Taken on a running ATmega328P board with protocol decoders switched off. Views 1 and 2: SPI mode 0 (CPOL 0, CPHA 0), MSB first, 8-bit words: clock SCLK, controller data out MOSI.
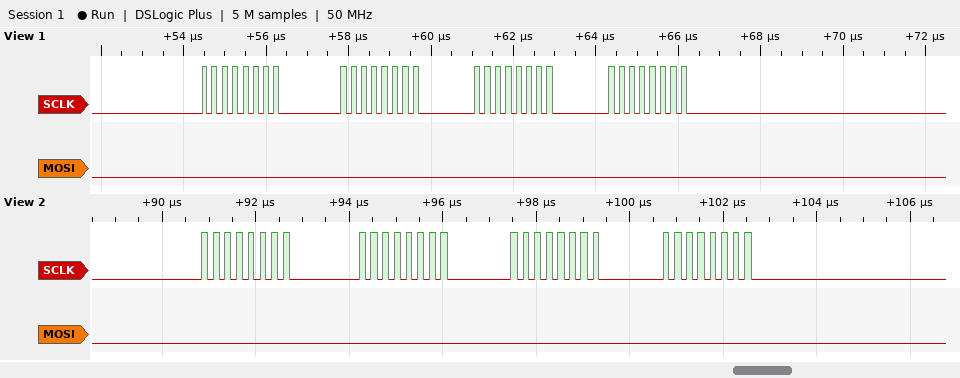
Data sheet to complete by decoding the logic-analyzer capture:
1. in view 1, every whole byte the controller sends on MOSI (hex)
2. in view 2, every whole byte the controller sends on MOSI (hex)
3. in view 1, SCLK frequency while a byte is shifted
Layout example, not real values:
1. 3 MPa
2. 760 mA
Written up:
1. 00 00 00 00
2. 00 00 00 00
3. 4 MHz
